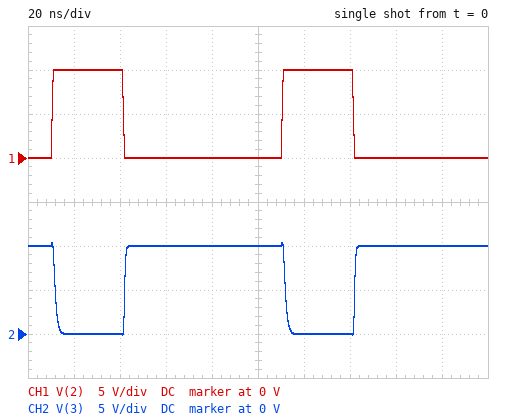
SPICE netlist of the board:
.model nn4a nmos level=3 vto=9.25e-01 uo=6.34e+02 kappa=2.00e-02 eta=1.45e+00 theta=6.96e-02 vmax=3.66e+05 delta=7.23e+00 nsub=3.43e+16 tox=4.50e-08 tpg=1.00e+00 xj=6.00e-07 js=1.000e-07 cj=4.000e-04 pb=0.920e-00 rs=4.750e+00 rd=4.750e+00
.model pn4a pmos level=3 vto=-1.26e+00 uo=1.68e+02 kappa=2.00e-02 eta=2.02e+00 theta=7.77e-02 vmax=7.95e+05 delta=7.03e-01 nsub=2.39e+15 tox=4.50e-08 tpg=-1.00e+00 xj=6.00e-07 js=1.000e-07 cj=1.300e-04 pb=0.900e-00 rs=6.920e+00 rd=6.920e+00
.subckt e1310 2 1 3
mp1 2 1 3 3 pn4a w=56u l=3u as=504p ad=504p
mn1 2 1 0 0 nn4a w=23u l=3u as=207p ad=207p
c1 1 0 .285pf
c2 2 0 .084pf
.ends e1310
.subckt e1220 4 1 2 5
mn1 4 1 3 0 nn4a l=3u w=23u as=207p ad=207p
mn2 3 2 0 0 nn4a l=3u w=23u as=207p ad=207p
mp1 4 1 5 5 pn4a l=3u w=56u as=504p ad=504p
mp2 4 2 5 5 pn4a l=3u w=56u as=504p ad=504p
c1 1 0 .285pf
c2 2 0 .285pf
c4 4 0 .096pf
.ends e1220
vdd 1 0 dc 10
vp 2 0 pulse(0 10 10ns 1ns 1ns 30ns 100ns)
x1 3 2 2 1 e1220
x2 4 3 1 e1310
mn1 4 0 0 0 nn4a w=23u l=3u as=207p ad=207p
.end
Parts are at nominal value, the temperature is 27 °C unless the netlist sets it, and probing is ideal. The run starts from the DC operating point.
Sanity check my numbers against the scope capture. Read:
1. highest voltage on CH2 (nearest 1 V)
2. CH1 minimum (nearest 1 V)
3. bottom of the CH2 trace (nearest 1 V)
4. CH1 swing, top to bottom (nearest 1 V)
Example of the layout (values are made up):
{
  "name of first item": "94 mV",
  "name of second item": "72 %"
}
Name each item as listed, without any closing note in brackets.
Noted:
{
  "highest voltage on CH2": "10 V",
  "CH1 minimum": "0 V",
  "bottom of the CH2 trace": "0 V",
  "CH1 swing, top to bottom": "10 V"
}
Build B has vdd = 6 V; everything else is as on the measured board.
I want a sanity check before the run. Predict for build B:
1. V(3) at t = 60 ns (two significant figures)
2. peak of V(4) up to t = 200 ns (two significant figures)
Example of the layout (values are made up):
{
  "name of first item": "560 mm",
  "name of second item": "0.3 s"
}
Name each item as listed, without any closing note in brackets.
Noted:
{
  "V(3) at t = 60 ns": "6.0 V",
  "peak of V(4) up to t = 200 ns": "6.3 V"
}
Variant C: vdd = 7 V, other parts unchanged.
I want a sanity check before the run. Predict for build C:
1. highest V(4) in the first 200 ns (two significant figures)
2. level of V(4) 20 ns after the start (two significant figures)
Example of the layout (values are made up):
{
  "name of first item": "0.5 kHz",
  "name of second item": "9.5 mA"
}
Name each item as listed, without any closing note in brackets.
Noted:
{
  "highest V(4) in the first 200 ns": "7.3 V",
  "level of V(4) 20 ns after the start": "7.0 V"
}
